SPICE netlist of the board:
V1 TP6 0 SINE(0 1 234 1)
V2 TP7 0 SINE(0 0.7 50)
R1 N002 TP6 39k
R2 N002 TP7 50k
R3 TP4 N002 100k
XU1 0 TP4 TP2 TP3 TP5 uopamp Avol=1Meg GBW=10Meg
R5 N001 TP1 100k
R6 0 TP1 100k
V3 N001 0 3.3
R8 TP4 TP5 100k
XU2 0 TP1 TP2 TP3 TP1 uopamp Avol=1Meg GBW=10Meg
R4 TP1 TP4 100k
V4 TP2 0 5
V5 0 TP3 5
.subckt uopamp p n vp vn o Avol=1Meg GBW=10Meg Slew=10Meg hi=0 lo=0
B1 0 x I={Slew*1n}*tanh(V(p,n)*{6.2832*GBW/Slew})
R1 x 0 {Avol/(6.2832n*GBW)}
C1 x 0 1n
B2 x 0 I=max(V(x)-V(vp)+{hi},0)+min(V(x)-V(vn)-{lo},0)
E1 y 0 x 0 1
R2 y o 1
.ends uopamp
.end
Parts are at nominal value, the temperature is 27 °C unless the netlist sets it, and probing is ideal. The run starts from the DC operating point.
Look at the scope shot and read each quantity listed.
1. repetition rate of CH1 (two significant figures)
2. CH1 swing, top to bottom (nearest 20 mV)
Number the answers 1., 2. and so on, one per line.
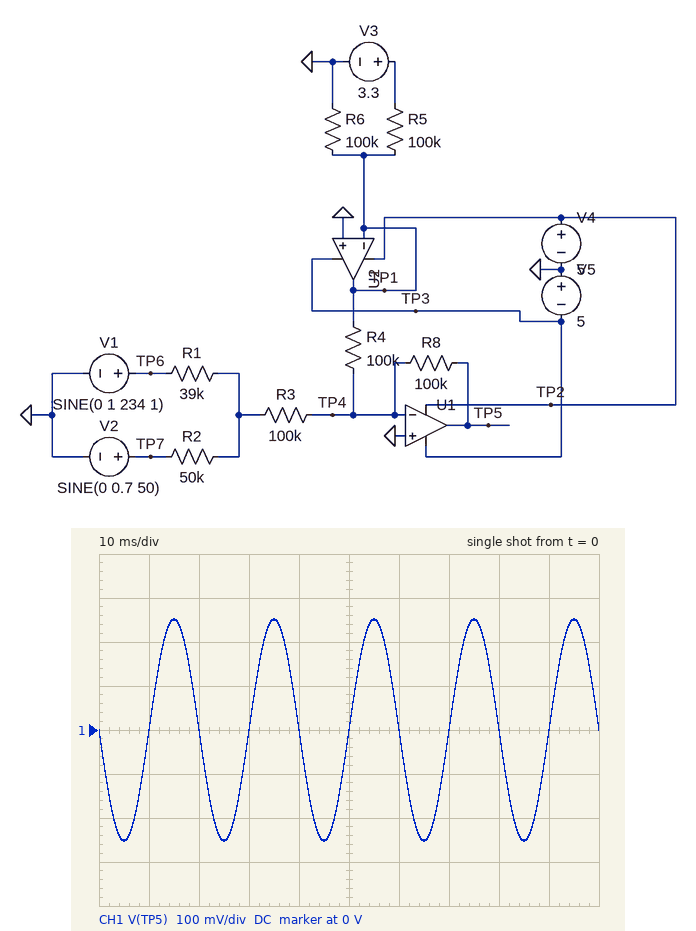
1. 50 Hz
2. 500 mV
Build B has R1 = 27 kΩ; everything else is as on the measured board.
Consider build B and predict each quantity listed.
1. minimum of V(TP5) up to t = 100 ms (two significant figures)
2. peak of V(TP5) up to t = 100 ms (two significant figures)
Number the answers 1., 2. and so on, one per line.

1. -210 mV
2. 210 mV
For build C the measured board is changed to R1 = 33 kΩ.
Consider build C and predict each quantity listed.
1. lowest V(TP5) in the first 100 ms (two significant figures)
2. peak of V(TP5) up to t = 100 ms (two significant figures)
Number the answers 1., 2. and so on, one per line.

1. -230 mV
2. 230 mV
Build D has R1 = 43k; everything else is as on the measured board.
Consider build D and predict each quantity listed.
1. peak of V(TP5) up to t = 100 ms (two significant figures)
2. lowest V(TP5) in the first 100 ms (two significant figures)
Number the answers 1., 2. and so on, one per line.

1. 260 mV
2. -260 mV
